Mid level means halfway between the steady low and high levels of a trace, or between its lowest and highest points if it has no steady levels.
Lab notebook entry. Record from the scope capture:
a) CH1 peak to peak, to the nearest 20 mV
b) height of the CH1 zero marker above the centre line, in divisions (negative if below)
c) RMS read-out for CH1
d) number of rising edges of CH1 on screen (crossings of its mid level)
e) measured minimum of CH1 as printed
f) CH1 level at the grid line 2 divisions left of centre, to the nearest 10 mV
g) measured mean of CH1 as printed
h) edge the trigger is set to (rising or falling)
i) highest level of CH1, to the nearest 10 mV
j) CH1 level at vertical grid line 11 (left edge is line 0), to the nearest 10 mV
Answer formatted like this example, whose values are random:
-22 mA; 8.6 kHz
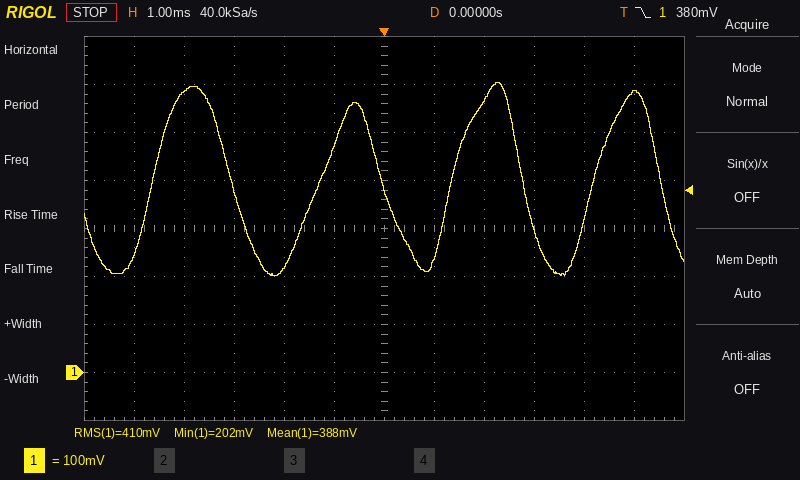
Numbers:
400 mV; -3.0 div; 410 mV; 4; 202 mV; 220 mV; 388 mV; falling; 600 mV; 580 mV
